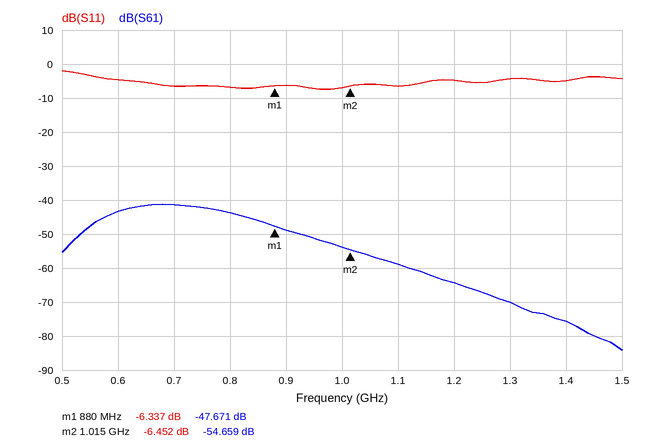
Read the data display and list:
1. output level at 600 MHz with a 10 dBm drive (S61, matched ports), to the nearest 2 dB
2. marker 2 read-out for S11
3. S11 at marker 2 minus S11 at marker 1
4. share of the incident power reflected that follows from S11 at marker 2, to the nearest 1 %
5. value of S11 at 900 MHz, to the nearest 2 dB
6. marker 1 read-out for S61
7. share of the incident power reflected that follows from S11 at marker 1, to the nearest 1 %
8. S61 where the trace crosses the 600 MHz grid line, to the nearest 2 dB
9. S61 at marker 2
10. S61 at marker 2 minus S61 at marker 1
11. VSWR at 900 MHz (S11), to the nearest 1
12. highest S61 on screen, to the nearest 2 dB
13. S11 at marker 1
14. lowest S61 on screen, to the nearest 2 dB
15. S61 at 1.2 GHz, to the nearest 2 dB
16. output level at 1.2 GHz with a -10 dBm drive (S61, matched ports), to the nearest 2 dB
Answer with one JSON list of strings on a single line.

["-34 dBm", "-6.452 dB", "-0.115 dB", "23 %", "-6 dB", "-47.671 dB", "23 %", "-44 dB", "-54.659 dB", "-6.988 dB", "3", "-42 dB", "-6.337 dB", "-84 dB", "-64 dB", "-74 dBm"]
